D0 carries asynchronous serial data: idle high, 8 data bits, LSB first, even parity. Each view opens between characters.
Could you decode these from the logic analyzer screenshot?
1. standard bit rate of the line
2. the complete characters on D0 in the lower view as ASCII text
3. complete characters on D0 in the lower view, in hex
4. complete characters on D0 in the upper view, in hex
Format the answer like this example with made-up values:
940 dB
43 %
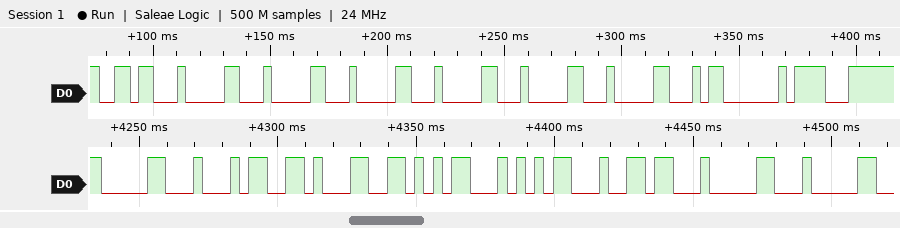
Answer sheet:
300 baud
"0415560"
30, 34, 31, 35, 35, 36, 30
36, 30, 30, 30, 30, 30, 30, 03, 8F
